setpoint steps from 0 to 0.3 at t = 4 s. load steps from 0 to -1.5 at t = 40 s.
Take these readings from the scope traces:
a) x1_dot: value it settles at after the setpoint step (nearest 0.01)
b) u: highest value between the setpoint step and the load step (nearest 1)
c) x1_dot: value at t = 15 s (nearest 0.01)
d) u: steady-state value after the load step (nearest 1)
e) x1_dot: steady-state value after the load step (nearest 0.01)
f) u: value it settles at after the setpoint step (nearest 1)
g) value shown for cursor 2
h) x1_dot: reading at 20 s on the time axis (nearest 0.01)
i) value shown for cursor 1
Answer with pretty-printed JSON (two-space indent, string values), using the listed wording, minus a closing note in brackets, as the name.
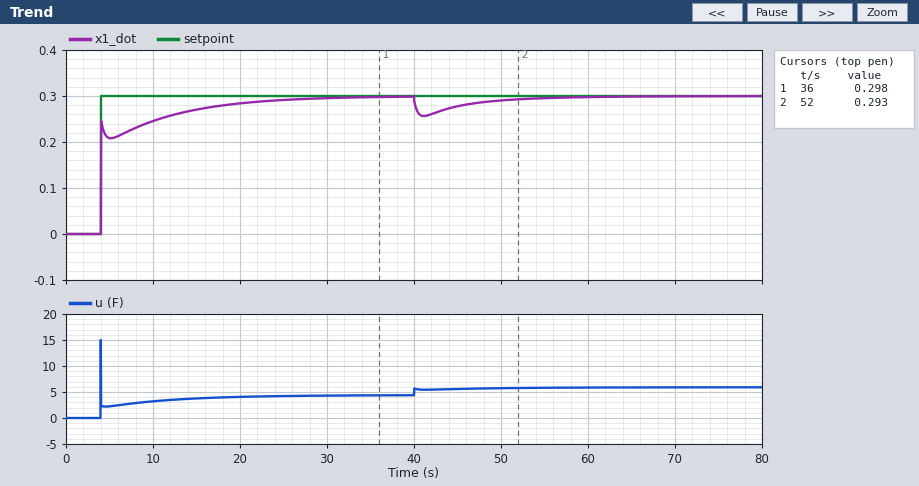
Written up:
{
  "x1_dot: value it settles at after the setpoint step": "0.30",
  "u: highest value between the setpoint step and the load step": "15",
  "x1_dot: value at t = 15 s": "0.27",
  "u: steady-state value after the load step": "6",
  "x1_dot: steady-state value after the load step": "0.30",
  "u: value it settles at after the setpoint step": "4",
  "value shown for cursor 2": "0.293",
  "x1_dot: reading at 20 s on the time axis": "0.28",
  "value shown for cursor 1": "0.298"
}
